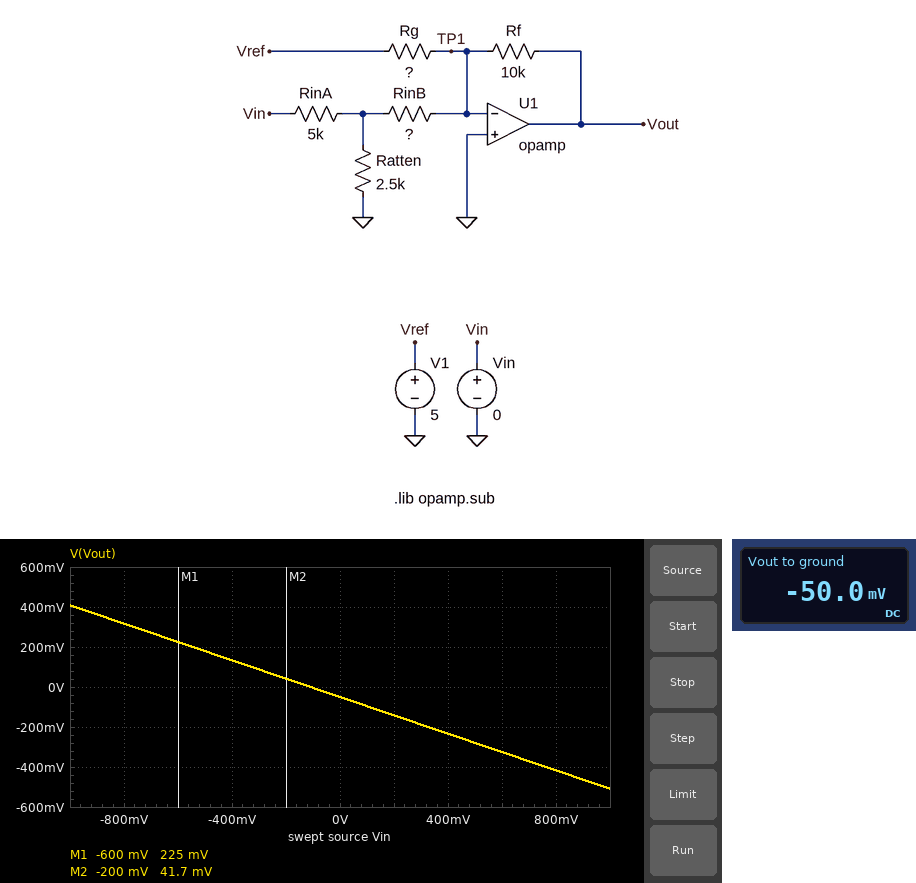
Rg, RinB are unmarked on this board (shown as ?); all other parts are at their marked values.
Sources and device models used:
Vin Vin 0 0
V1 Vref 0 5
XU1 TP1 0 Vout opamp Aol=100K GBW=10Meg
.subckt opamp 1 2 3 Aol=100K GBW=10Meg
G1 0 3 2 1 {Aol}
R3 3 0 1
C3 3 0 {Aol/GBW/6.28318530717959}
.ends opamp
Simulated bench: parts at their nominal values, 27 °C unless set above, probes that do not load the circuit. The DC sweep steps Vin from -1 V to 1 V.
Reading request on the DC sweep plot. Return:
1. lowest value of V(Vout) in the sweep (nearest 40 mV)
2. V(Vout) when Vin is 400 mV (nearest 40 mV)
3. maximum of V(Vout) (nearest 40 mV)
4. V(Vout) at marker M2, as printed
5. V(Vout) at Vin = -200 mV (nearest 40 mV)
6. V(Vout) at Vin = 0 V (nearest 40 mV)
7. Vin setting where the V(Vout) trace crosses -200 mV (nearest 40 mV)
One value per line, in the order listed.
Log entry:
-520 mV
-240 mV
400 mV
41.7 mV
40 mV
-40 mV
320 mV
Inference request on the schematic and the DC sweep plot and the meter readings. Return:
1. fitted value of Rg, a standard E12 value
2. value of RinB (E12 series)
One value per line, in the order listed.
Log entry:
1 MΩ
5.6 kΩ
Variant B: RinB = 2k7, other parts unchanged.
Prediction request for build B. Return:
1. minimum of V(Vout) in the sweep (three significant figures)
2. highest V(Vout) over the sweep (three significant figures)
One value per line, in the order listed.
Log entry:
-813 mV
713 mV
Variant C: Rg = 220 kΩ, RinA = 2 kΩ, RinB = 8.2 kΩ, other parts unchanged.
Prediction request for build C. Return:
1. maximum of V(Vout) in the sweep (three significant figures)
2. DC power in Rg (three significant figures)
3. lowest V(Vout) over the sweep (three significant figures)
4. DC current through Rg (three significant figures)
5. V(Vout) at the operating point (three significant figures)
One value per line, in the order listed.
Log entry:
369 mV
114 µW
-824 mV
22.7 µA
-227 mV
